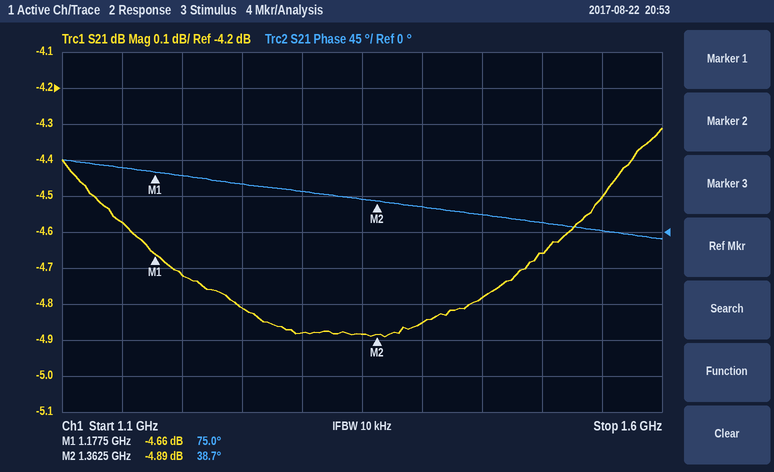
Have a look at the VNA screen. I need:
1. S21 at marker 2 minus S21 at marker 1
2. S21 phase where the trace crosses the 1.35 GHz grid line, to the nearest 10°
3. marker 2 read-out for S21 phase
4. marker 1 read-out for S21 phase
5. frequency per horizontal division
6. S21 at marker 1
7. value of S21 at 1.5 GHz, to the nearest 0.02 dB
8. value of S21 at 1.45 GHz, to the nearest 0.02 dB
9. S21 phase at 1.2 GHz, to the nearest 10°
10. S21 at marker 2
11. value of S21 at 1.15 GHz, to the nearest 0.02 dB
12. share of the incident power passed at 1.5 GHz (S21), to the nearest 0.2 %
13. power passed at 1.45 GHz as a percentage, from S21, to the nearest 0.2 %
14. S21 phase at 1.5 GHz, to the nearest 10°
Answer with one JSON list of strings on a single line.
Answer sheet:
["-0.23 dB", "40°", "38.7°", "75.0°", "50 MHz", "-4.66 dB", "-4.66 dB", "-4.78 dB", "70°", "-4.89 dB", "-4.58 dB", "34.2 %", "33.2 %", "10°"]
